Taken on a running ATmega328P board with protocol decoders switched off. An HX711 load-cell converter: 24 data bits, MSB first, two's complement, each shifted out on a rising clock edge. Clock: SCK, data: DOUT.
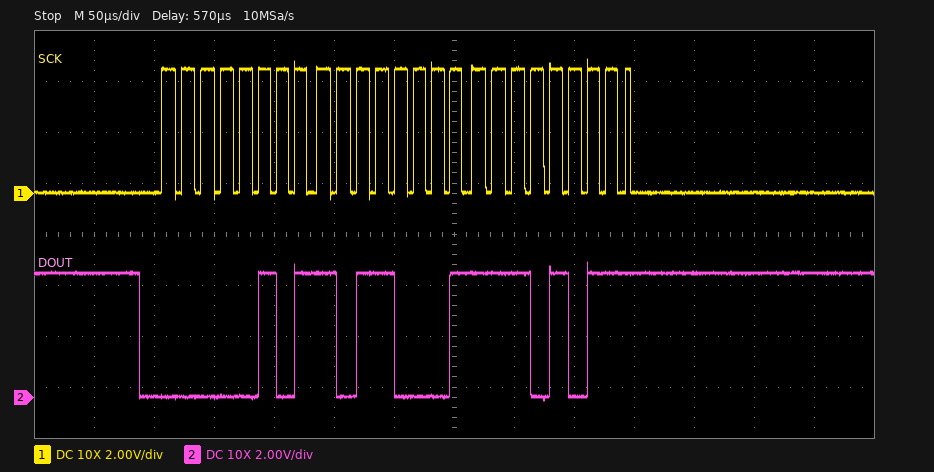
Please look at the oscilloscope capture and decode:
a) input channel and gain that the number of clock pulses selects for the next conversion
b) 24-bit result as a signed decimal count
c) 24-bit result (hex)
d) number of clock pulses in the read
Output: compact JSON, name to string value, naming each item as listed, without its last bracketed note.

{"input channel and gain that the number of clock pulses selects for the next conversion": "channel A, gain 128", "24-bit result as a signed decimal count": "373227", "24-bit result": "0x05B1EB", "number of clock pulses in the read": "25"}
